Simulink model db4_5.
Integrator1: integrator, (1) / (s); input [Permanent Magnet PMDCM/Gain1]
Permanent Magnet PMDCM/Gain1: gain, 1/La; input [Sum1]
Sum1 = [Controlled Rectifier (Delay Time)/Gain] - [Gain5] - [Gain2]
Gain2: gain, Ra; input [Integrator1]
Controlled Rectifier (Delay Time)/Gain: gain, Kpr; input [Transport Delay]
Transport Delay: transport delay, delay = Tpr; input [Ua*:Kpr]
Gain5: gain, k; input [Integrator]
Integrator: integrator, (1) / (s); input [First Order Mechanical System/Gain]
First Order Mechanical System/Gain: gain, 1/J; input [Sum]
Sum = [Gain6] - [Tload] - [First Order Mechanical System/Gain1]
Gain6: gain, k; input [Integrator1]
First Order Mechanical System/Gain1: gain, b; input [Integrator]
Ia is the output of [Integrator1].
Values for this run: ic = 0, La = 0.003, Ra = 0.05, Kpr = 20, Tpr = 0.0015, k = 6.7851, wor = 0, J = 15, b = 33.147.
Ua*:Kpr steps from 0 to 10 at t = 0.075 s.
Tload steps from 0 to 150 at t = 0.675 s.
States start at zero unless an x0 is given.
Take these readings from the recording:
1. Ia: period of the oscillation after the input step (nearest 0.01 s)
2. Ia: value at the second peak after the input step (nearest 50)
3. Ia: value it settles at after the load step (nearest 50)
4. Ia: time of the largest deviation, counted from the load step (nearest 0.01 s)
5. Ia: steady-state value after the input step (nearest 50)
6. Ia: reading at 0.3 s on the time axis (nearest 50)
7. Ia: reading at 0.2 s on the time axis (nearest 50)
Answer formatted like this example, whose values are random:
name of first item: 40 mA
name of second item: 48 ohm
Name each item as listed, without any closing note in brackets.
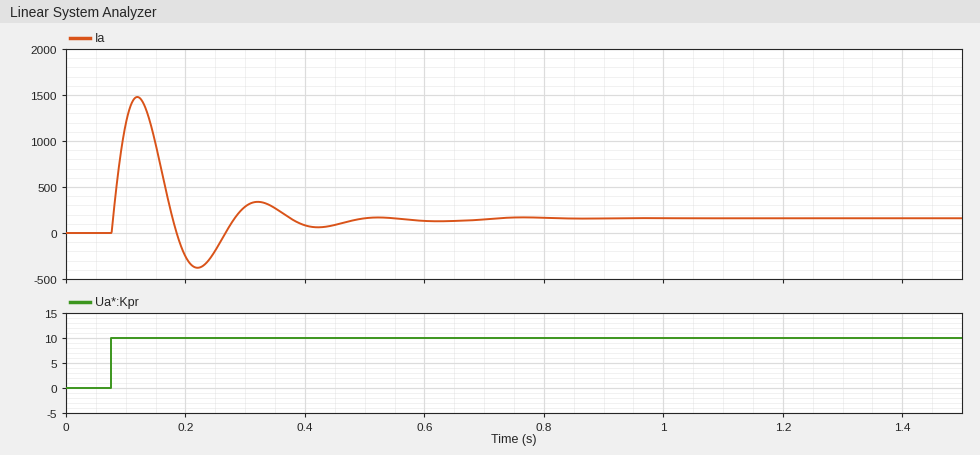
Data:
Ia: period of the oscillation after the input step: 0.20 s
Ia: value at the second peak after the input step: 350
Ia: value it settles at after the load step: 150
Ia: time of the largest deviation, counted from the load step: 0.09 s
Ia: steady-state value after the input step: 150
Ia: reading at 0.3 s on the time axis: 300
Ia: reading at 0.2 s on the time axis: -250
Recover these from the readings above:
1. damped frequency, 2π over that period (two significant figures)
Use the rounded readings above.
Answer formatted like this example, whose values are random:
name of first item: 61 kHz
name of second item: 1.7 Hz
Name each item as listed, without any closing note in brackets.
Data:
damped frequency, 2π over that period: 31 rad/s
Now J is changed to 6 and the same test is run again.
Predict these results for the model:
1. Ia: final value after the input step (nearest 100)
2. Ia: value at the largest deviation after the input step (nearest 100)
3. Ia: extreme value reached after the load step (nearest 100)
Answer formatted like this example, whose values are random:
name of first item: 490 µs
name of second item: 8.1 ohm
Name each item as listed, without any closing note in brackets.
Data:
Ia: final value after the input step: 100
Ia: value at the largest deviation after the input step: 1100
Ia: extreme value reached after the load step: 200
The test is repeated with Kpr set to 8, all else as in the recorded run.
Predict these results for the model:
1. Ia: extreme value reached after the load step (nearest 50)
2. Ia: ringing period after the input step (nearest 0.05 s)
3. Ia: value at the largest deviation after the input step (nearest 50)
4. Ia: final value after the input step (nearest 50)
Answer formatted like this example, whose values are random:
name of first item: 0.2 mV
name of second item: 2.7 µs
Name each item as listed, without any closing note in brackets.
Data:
Ia: extreme value reached after the load step: 100
Ia: ringing period after the input step: 0.20 s
Ia: value at the largest deviation after the input step: 600
Ia: final value after the input step: 50
